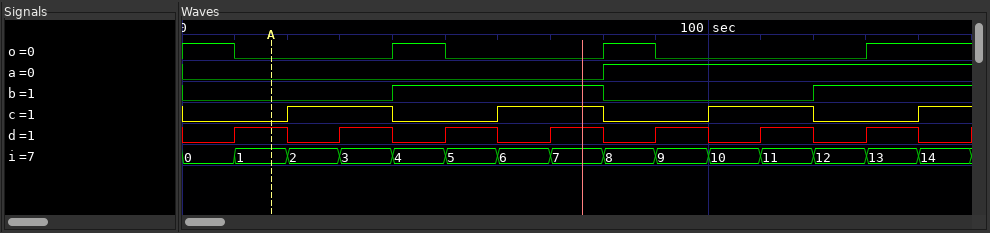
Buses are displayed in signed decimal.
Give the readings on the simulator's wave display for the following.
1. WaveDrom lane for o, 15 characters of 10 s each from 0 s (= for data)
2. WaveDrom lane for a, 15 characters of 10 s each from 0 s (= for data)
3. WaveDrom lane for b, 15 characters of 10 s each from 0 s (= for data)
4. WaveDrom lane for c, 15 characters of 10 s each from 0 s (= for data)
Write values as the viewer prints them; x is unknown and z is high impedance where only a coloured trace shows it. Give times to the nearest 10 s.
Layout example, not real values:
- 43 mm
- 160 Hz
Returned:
- {name: 'o', wave: '10..10..10...1.'}
- {name: 'a', wave: '0.......1......'}
- {name: 'b', wave: '0...1...0...1..'}
- {name: 'c', wave: '0.1.0.1.0.1.0.1'}
